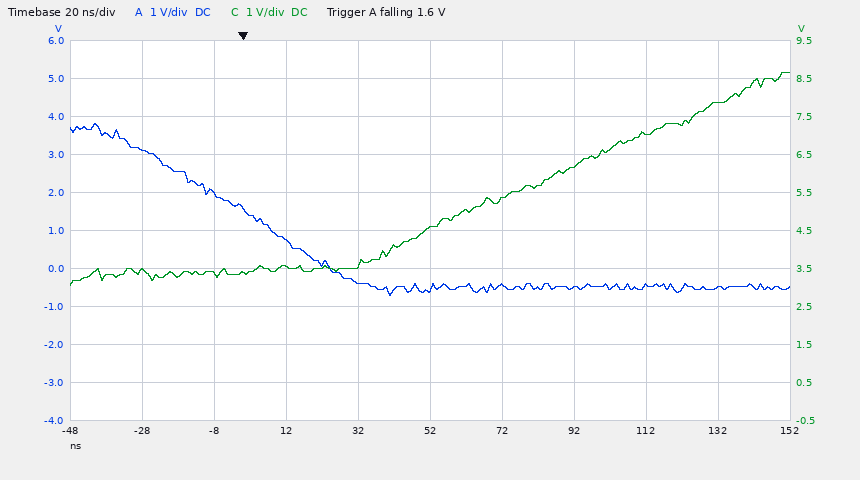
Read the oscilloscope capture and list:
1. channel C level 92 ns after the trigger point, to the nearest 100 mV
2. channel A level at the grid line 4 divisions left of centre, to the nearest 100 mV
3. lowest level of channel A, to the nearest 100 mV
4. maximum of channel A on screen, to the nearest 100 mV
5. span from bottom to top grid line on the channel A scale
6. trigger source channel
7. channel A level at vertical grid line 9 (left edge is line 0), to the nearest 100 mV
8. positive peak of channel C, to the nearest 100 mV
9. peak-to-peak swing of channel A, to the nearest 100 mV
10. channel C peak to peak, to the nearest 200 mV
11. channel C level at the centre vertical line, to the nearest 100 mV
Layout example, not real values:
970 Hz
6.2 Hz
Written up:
6.2 V
3.1 V
-700 mV
3.8 V
10 V
channel A
-500 mV
8.7 V
4.5 V
5.6 V
4.6 V
